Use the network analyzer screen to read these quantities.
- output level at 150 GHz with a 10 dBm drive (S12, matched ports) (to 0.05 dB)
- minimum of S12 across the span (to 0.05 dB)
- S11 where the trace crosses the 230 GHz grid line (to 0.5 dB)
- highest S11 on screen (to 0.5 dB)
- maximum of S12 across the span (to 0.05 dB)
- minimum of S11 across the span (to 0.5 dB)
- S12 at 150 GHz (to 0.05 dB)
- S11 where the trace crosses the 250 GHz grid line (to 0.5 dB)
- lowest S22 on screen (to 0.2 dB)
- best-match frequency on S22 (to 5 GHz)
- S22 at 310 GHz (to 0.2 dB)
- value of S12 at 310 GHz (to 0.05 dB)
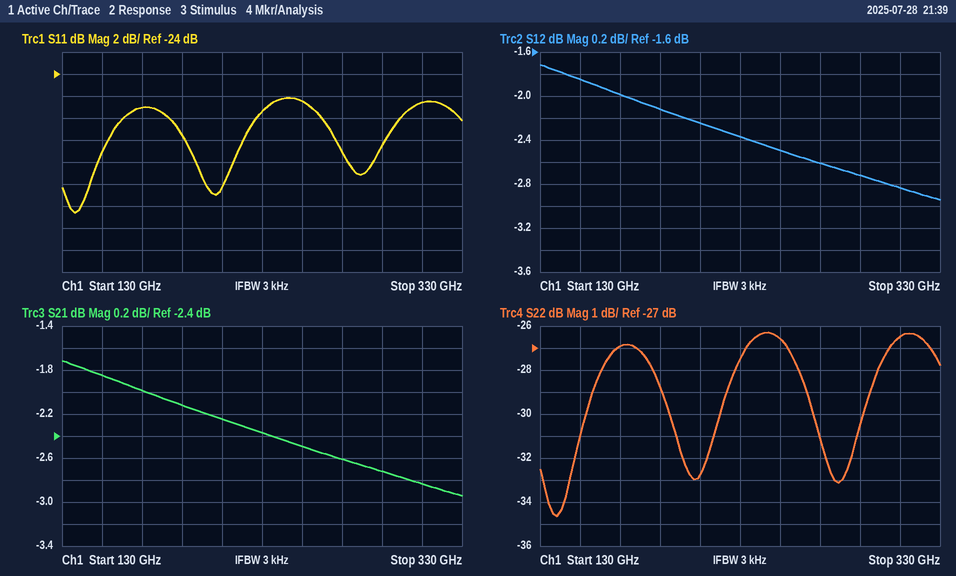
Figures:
8.15 dBm
-2.95 dB
-27.5 dB
-26.0 dB
-1.70 dB
-36.5 dB
-1.85 dB
-26.5 dB
-34.6 dB
140 GHz
-26.4 dB
-2.85 dB
